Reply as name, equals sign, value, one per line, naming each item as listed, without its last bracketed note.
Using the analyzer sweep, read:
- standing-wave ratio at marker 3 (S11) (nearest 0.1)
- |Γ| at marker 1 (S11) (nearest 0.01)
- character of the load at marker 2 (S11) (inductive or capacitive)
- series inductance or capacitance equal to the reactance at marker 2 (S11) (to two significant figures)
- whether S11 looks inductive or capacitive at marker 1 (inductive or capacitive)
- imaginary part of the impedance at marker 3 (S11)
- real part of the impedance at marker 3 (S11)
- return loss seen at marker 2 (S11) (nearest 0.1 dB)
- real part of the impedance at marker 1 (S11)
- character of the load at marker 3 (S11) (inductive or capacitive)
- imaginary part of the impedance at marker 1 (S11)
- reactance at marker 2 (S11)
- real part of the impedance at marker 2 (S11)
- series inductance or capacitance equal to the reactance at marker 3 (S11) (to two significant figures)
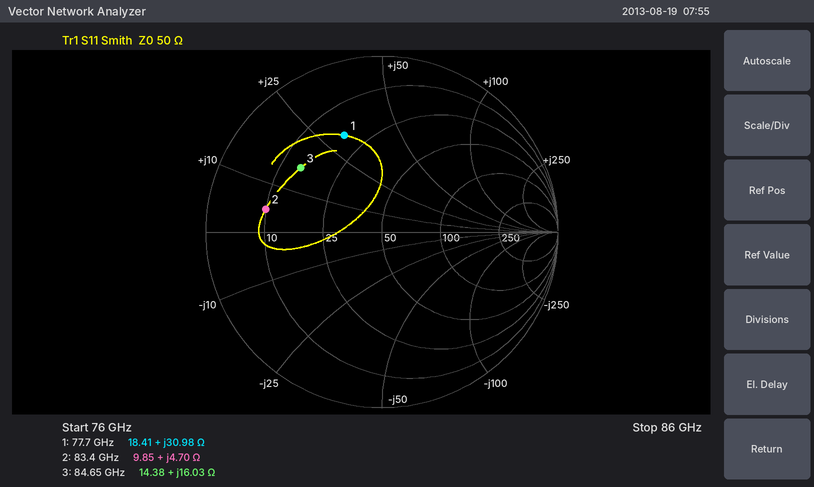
standing-wave ratio at marker 3 (S11) = 3.9
|Γ| at marker 1 (S11) = 0.59
character of the load at marker 2 (S11) = inductive
series inductance or capacitance equal to the reactance at marker 2 (S11) = 9.0 pH
whether S11 looks inductive or capacitive at marker 1 = inductive
imaginary part of the impedance at marker 3 = +16.03 Ω
real part of the impedance at marker 3 = 14.38 Ω
return loss seen at marker 2 (S11) = 3.4 dB
real part of the impedance at marker 1 = 18.41 Ω
character of the load at marker 3 (S11) = inductive
imaginary part of the impedance at marker 1 = +30.98 Ω
reactance at marker 2 = +4.70 Ω
real part of the impedance at marker 2 = 9.85 Ω
series inductance or capacitance equal to the reactance at marker 3 (S11) = 30 pH
